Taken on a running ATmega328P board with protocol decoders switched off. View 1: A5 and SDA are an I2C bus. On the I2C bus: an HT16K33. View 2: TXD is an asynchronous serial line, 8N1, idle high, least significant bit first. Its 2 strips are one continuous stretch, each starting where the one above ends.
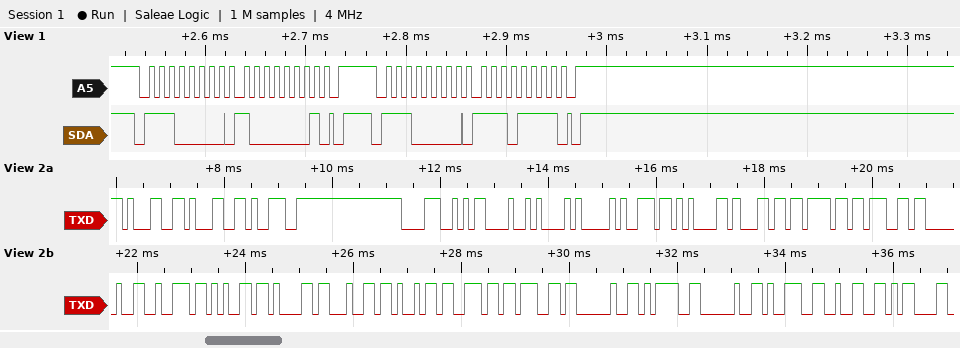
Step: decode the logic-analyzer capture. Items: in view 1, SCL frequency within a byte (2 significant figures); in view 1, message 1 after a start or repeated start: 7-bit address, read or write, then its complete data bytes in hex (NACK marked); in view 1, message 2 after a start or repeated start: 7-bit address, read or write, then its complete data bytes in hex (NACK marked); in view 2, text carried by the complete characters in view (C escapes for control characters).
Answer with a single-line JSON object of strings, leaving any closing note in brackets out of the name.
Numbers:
{"in view 1, SCL frequency within a byte": "100 kHz", "in view 1, message 1 after a start or repeated start: 7-bit address, read or write, then its complete data bytes in hex": "0x70 write: 81", "in view 1, message 2 after a start or repeated start: 7-bit address, read or write, then its complete data bytes in hex": "0x70 write: EF", "in view 2, text carried by the complete characters in view": "\"1198\\r\\nAnalog reading = 92\\r\""}
